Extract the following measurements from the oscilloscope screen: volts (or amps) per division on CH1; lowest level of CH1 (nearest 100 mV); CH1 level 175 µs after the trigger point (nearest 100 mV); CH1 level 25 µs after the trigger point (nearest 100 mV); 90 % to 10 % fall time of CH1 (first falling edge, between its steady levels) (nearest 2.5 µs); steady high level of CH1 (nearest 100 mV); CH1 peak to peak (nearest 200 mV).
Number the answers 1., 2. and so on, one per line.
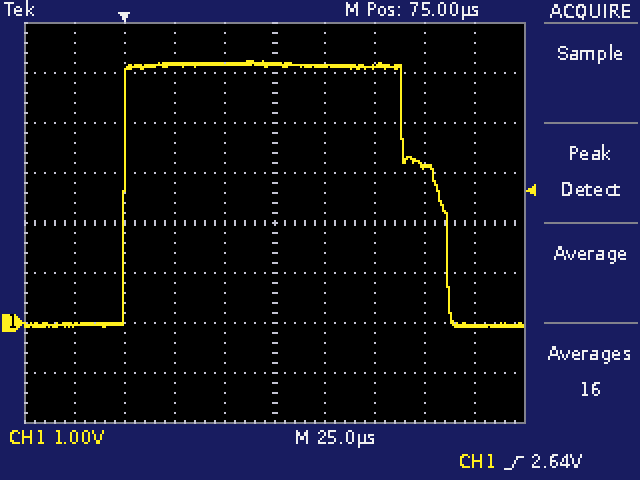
1. 1 V
2. -100 mV
3. -100 mV
4. 5.2 V
5. 25.0 µs
6. 5.2 V
7. 5.4 V
